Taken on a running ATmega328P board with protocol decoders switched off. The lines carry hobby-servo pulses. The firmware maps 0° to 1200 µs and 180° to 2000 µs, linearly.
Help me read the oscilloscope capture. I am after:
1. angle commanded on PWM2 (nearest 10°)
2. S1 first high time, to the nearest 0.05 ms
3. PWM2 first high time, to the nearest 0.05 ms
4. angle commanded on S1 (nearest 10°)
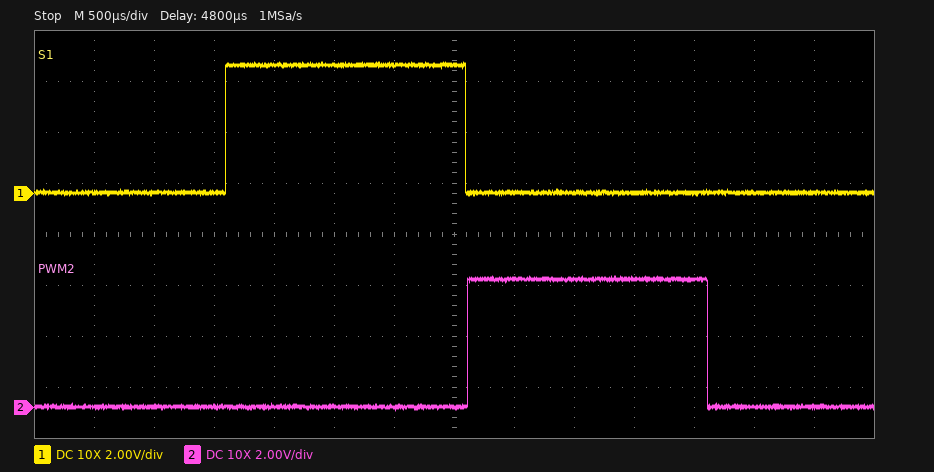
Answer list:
180°
2.00 ms
2.00 ms
180°
